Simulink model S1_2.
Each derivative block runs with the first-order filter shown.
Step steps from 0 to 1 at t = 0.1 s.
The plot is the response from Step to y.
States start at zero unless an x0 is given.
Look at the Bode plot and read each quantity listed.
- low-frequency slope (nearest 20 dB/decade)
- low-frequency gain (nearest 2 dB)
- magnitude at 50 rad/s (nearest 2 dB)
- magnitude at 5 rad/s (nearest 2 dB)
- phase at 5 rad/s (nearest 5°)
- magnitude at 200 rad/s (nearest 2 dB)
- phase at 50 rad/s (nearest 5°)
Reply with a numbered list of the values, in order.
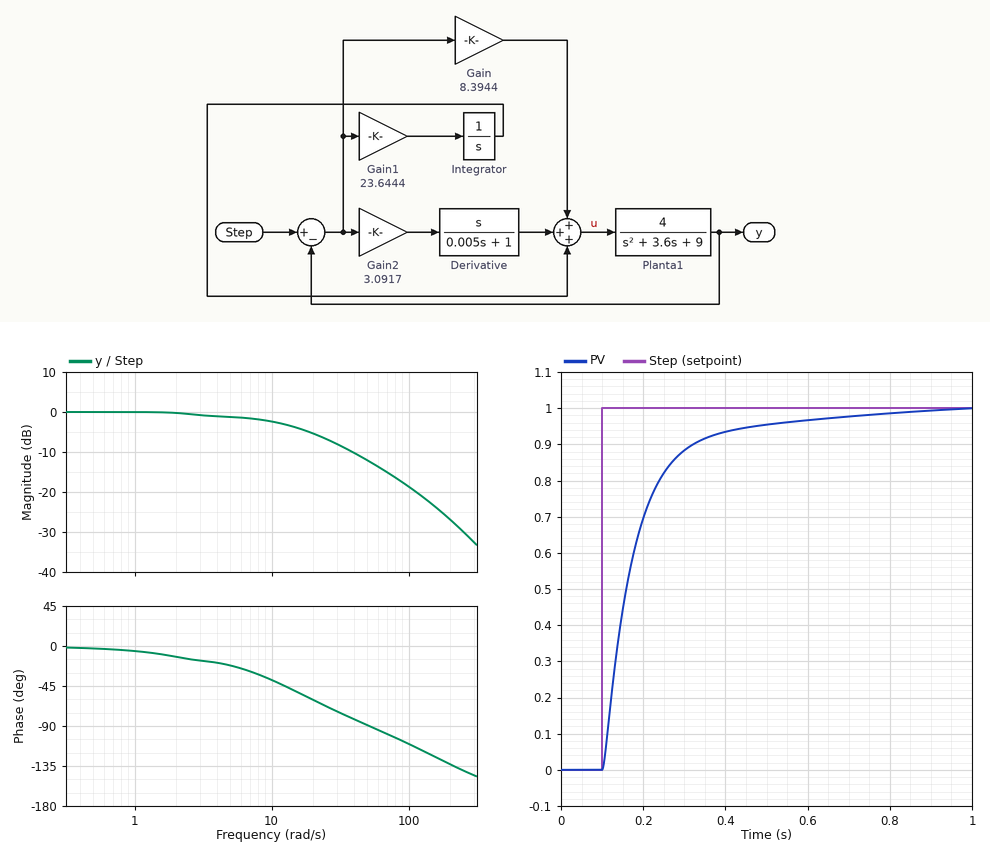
1. 0 dB/decade
2. 0 dB
3. -12 dB
4. -2 dB
5. -20°
6. -26 dB
7. -90°
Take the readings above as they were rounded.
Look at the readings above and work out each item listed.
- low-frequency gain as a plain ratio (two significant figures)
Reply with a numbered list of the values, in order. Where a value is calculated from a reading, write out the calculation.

1. 10^(0 / 20) = 1.0
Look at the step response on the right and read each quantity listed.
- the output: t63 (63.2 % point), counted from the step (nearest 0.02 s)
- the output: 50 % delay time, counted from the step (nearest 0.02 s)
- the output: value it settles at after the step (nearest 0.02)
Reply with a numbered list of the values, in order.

1. 0.08 s
2. 0.06 s
3. 1.00
